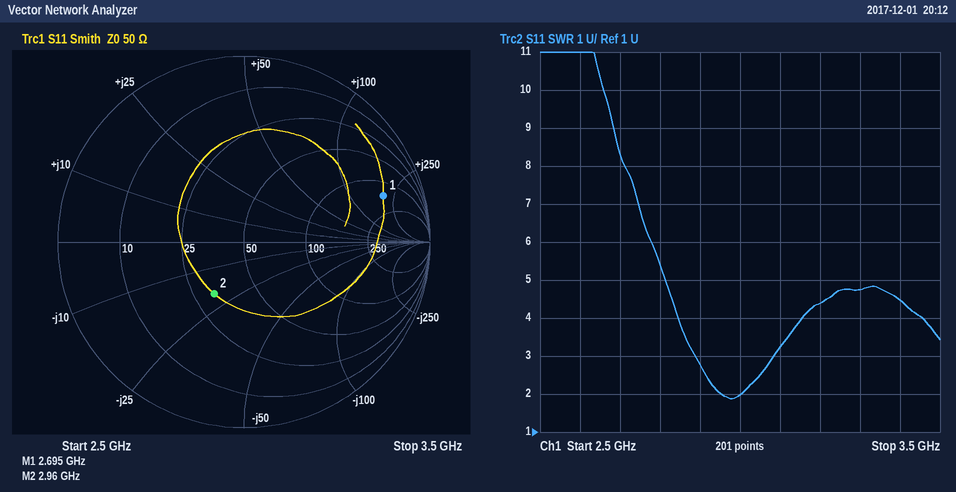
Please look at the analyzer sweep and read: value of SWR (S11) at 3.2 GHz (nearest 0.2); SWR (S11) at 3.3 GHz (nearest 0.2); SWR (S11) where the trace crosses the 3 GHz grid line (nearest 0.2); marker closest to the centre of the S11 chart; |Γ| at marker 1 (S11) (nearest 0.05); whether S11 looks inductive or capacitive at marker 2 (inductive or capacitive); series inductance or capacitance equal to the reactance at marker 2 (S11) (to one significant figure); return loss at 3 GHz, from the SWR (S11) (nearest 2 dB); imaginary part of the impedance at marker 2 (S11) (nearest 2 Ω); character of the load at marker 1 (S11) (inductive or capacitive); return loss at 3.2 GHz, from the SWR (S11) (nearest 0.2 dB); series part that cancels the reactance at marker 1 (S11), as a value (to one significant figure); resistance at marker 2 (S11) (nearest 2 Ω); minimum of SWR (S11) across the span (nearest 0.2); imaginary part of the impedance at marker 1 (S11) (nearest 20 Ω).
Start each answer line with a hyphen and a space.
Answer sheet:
- 4.4
- 4.8
- 2.0
- marker 2
- 0.80
- capacitive
- 3 pF
- 10 dB
- -20 Ω
- inductive
- 4.0 dB
- 300 fF
- 32 Ω
- 1.8
- +200 Ω
